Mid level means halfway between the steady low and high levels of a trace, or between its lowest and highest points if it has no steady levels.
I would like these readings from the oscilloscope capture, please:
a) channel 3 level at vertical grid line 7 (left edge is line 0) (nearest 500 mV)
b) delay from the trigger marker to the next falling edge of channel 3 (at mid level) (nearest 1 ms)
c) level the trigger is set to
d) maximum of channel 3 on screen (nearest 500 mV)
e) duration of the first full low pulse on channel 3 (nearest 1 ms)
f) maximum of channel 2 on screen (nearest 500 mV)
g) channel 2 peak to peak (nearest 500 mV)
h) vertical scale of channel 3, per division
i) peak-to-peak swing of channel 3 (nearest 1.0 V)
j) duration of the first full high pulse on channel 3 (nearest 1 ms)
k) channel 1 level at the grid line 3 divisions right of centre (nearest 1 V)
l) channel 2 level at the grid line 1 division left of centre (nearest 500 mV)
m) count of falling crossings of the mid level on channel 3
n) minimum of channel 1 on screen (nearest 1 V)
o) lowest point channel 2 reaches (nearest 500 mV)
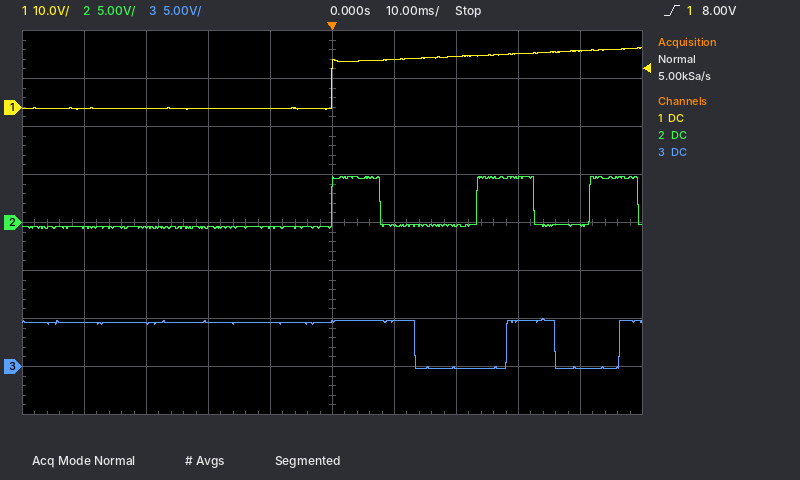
0.0 V
13 ms
8.00 V
5.0 V
15 ms
5.0 V
5.5 V
5 V
5.0 V
8 ms
11 V
-500 mV
2
0 V
-500 mV
